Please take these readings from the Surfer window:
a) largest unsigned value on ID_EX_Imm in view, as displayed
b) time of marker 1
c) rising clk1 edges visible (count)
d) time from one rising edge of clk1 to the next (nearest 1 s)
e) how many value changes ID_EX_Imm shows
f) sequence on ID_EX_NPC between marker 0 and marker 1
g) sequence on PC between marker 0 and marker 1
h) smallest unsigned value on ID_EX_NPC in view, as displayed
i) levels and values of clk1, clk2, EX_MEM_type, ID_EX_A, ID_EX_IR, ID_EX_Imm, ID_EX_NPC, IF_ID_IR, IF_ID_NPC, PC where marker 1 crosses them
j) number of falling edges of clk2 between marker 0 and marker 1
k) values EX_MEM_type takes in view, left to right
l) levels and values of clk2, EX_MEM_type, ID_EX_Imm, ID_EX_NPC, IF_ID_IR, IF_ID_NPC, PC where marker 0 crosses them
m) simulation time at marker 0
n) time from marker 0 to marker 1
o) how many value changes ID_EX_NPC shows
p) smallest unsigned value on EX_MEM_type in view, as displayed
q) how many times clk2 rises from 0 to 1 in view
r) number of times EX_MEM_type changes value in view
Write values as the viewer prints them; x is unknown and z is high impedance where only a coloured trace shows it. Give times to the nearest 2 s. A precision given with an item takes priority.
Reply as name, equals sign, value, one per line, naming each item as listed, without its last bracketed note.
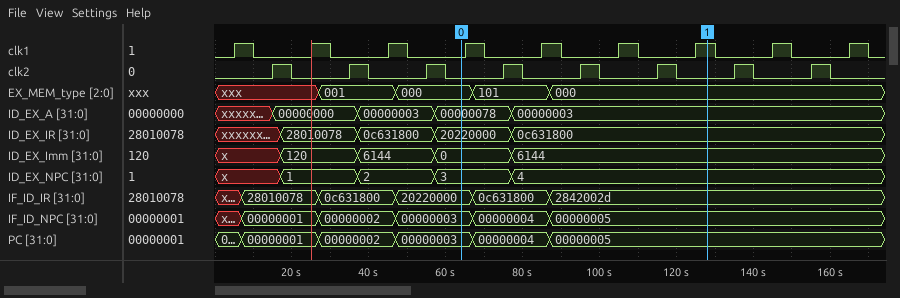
largest unsigned value on ID_EX_Imm in view, as displayed = 6144
time of marker 1 = 128 s
rising clk1 edges visible = 9
time from one rising edge of clk1 to the next = 20 s
how many value changes ID_EX_Imm shows = 4
sequence on ID_EX_NPC between marker 0 and marker 1 = 3, 4
sequence on PC between marker 0 and marker 1 = 00000003, 00000004, 00000005
smallest unsigned value on ID_EX_NPC in view, as displayed = 1
levels and values of clk1, clk2, EX_MEM_type, ID_EX_A, ID_EX_IR, ID_EX_Imm, ID_EX_NPC, IF_ID_IR, IF_ID_NPC, PC where marker 1 crosses them = clk1=1, clk2=0, EX_MEM_type=000, ID_EX_A=00000003, ID_EX_IR=0c631800, ID_EX_Imm=6144, ID_EX_NPC=4, IF_ID_IR=2842002d, IF_ID_NPC=00000005, PC=00000005
number of falling edges of clk2 between marker 0 and marker 1 = 3
values EX_MEM_type takes in view, left to right = xxx, 001, 000, 101, 000
levels and values of clk2, EX_MEM_type, ID_EX_Imm, ID_EX_NPC, IF_ID_IR, IF_ID_NPC, PC where marker 0 crosses them = clk2=0, EX_MEM_type=000, ID_EX_Imm=0, ID_EX_NPC=3, IF_ID_IR=20220000, IF_ID_NPC=00000003, PC=00000003
simulation time at marker 0 = 64 s
time from marker 0 to marker 1 = 64 s
how many value changes ID_EX_NPC shows = 4
smallest unsigned value on EX_MEM_type in view, as displayed = 000
how many times clk2 rises from 0 to 1 in view = 8
number of times EX_MEM_type changes value in view = 4
